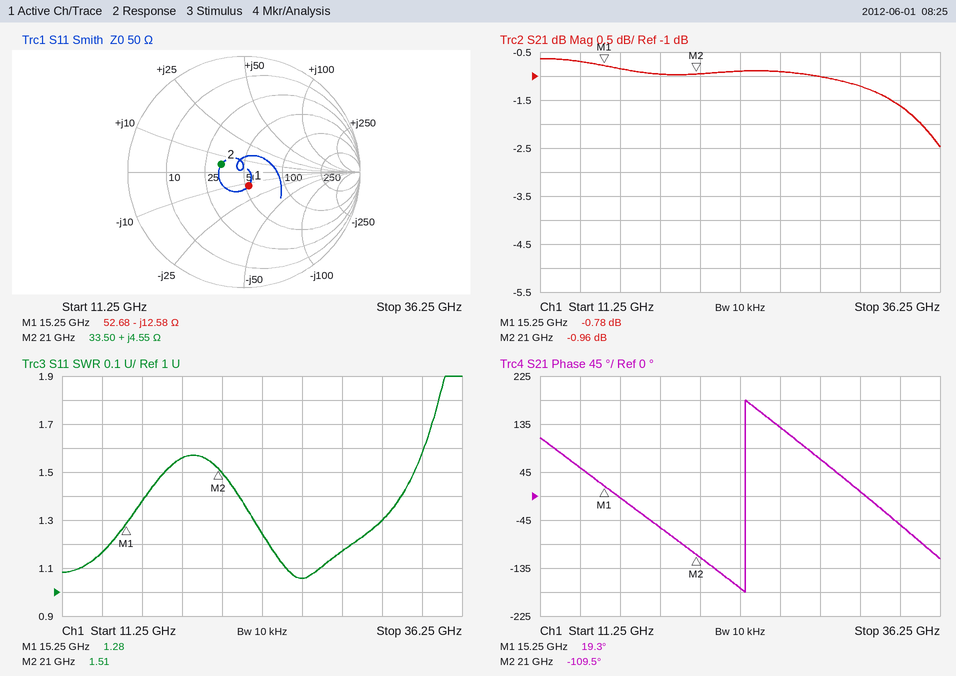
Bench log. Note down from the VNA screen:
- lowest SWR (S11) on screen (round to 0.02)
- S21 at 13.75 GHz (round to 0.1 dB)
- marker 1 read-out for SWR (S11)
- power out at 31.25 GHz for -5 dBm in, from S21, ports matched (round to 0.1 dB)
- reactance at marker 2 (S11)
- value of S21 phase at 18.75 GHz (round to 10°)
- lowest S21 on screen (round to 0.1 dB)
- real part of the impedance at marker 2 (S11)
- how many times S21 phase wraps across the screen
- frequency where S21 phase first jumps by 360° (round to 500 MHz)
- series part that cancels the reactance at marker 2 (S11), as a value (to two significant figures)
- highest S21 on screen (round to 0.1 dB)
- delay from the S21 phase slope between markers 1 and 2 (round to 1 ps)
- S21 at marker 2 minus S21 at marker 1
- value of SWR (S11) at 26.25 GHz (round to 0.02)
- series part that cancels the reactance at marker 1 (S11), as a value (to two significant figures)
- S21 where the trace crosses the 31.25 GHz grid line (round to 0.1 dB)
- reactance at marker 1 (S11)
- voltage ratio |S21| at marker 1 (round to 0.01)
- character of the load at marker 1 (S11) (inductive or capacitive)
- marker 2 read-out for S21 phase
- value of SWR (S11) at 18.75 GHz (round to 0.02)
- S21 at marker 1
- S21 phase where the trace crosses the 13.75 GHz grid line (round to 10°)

1.06
-0.7 dB
1.28
-6.2 dBm
+4.55 Ω
-60°
-2.5 dB
33.50 Ω
1
24.0 GHz
1.7 pF
-0.6 dB
62 ps
-0.18 dB
1.06
130 pH
-1.2 dB
-12.58 Ω
0.91
capacitive
-109.5°
1.56
-0.78 dB
50°
